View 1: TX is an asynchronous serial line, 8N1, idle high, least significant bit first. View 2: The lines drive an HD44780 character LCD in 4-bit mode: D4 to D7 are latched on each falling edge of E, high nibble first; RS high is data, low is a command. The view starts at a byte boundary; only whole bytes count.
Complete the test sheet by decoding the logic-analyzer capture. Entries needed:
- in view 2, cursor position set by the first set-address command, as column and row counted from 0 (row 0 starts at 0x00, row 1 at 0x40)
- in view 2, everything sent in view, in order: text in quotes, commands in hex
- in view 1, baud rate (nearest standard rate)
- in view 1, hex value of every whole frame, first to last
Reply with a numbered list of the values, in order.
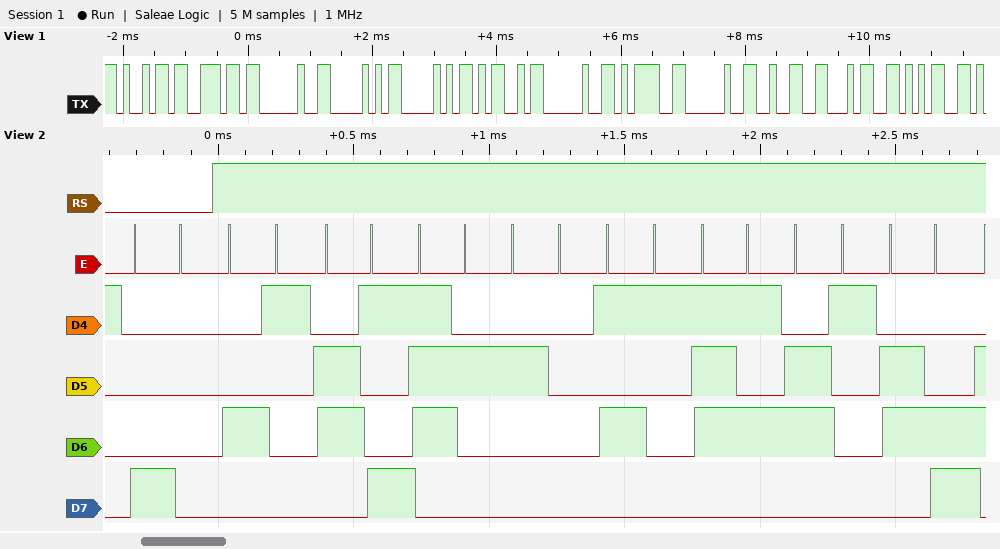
1. column 0, row 0
2. 0x80 "Air Qual"
3. 9600 baud
4. 0x69 0x6E 0x20 0x50 0x50 0x4D 0x20 0x3D 0x20 0x32 0x34 0x35
